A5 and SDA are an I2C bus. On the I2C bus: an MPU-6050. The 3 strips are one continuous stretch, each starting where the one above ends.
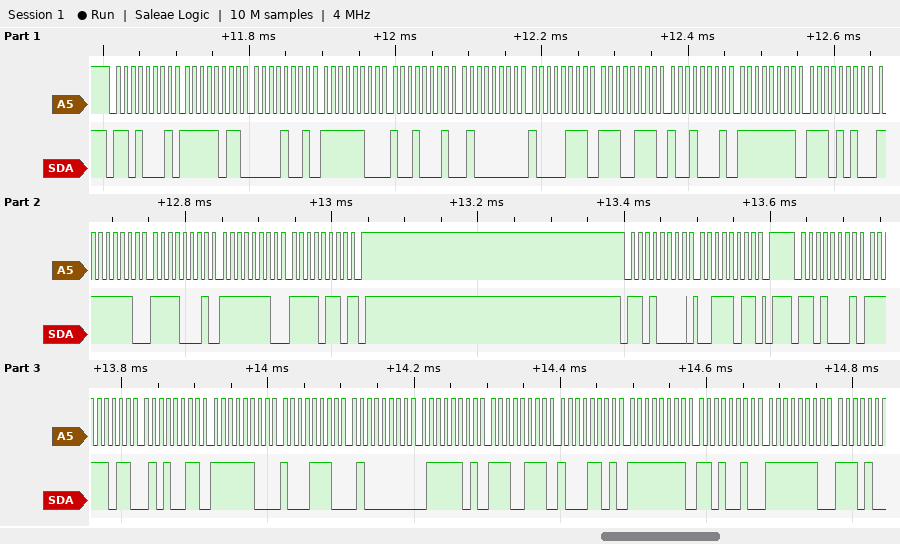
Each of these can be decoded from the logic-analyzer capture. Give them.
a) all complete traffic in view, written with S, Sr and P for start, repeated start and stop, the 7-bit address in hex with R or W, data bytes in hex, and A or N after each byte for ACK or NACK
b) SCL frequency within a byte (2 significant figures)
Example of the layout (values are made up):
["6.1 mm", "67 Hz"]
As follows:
["S 68R A FB A 09 A FC A 91 A 40 A 87 A E7 A 91 A FF A EA A FE A F1 A FE A F6 N P S 68W A 3B A P S 68R A FB A 53 A FC A 8E A 40 A 7D A E7 A 8D A FF A D2 A FE A", "100 kHz"]
